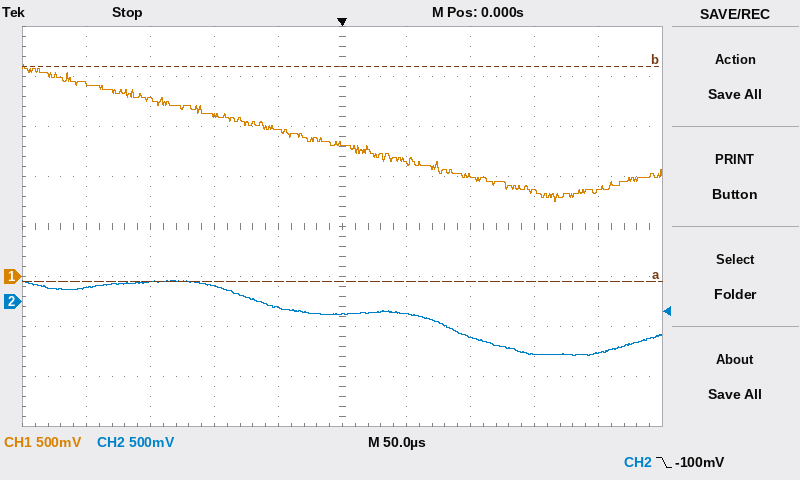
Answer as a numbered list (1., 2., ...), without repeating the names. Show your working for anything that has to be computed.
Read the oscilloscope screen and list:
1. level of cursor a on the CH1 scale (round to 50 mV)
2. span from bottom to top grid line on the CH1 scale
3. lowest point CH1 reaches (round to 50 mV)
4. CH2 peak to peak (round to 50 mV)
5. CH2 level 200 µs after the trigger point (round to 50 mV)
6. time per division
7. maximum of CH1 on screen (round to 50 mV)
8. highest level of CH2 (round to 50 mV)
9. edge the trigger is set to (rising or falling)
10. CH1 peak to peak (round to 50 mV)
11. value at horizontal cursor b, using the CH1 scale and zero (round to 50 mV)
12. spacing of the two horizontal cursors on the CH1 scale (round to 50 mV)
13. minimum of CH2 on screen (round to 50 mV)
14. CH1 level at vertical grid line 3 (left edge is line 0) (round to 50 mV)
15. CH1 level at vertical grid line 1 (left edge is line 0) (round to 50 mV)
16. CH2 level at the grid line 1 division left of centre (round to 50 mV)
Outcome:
1. -50 mV
2. 4 V
3. 750 mV
4. 200 mV − (-550 mV) = 750 mV
5. -500 mV
6. 50 µs
7. 2.10 V
8. 200 mV
9. falling
10. 2.10 V − (750 mV) = 1.35 V
11. 2.10 V
12. 2.15 V
13. -550 mV
14. 1.60 V
15. 1.95 V
16. -50 mV
